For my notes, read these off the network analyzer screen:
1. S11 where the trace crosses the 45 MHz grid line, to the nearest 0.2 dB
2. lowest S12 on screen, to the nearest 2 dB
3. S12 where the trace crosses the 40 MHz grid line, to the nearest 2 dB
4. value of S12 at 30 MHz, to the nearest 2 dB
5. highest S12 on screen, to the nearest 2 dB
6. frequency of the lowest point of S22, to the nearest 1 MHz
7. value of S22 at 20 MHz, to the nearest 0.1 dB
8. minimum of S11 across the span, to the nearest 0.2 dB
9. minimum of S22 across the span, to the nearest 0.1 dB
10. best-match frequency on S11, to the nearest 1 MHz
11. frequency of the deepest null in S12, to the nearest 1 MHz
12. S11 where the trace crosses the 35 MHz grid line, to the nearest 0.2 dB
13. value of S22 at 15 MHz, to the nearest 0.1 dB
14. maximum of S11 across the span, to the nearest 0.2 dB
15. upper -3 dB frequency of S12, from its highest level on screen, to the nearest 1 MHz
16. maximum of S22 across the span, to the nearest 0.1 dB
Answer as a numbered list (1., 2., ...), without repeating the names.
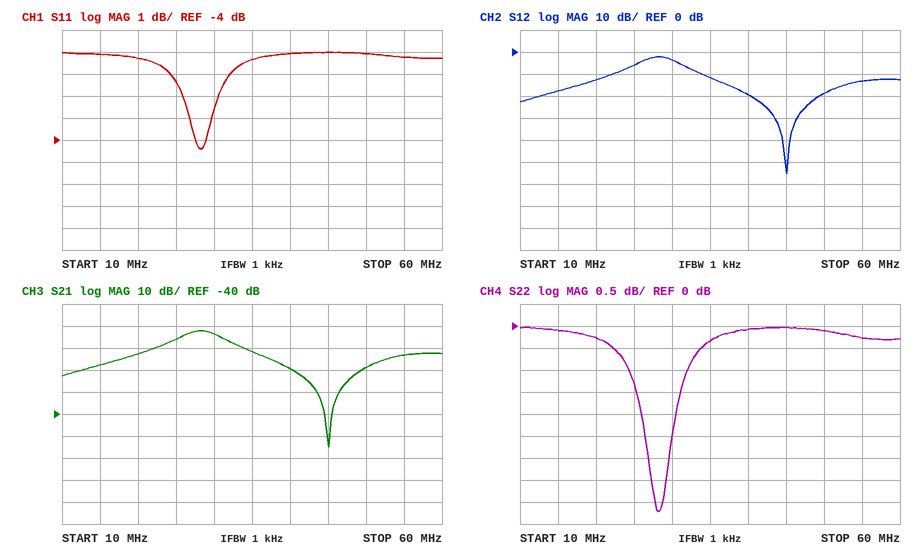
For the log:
1. 0.0 dB
2. -56 dB
3. -20 dB
4. -4 dB
5. -2 dB
6. 28 MHz
7. -0.3 dB
8. -4.4 dB
9. -4.2 dB
10. 28 MHz
11. 45 MHz
12. -0.4 dB
13. -0.1 dB
14. 0.0 dB
15. 31 MHz
16. 0.0 dB
